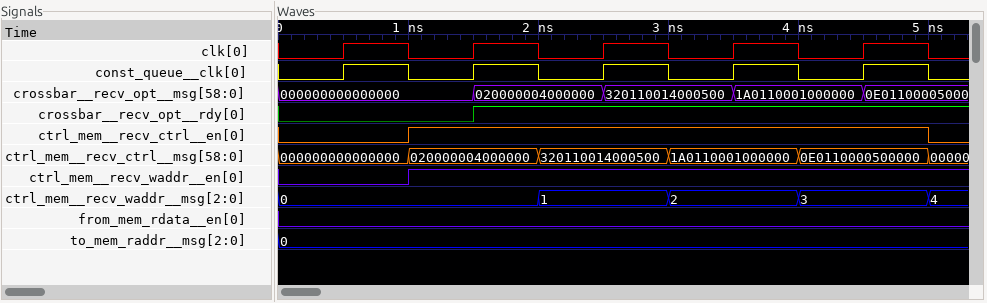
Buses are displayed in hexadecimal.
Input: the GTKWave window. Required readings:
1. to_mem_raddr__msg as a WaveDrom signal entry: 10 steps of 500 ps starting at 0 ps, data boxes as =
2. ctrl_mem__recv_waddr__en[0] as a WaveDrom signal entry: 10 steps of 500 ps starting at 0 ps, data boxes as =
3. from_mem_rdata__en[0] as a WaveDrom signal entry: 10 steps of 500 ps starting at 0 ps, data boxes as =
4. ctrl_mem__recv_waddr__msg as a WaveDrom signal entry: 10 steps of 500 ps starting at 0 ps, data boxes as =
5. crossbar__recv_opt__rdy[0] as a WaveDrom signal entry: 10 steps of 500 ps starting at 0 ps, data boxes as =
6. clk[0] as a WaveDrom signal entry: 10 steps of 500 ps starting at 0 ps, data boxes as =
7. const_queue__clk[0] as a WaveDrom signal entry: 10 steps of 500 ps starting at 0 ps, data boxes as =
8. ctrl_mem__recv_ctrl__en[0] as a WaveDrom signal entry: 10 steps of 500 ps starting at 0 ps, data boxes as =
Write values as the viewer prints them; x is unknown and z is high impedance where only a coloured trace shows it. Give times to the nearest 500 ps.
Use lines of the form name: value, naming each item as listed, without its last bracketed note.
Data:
to_mem_raddr__msg as a WaveDrom signal entry: 10 steps of 500 ps starting at 0 ps, data boxes as =: {name: 'to_mem_raddr__msg', wave: '=.........', data: '0'}
ctrl_mem__recv_waddr__en[0] as a WaveDrom signal entry: 10 steps of 500 ps starting at 0 ps, data boxes as =: {name: 'ctrl_mem__recv_waddr__en[0]', wave: '0.1.......'}
from_mem_rdata__en[0] as a WaveDrom signal entry: 10 steps of 500 ps starting at 0 ps, data boxes as =: {name: 'from_mem_rdata__en[0]', wave: '0.........'}
ctrl_mem__recv_waddr__msg as a WaveDrom signal entry: 10 steps of 500 ps starting at 0 ps, data boxes as =: {name: 'ctrl_mem__recv_waddr__msg', wave: '=...=.=.=.', data: '0 1 2 3'}
crossbar__recv_opt__rdy[0] as a WaveDrom signal entry: 10 steps of 500 ps starting at 0 ps, data boxes as =: {name: 'crossbar__recv_opt__rdy[0]', wave: '0..1......'}
clk[0] as a WaveDrom signal entry: 10 steps of 500 ps starting at 0 ps, data boxes as =: {name: 'clk[0]', wave: '0101010101'}
const_queue__clk[0] as a WaveDrom signal entry: 10 steps of 500 ps starting at 0 ps, data boxes as =: {name: 'const_queue__clk[0]', wave: '0101010101'}
ctrl_mem__recv_ctrl__en[0] as a WaveDrom signal entry: 10 steps of 500 ps starting at 0 ps, data boxes as =: {name: 'ctrl_mem__recv_ctrl__en[0]', wave: '0.1.......'}
